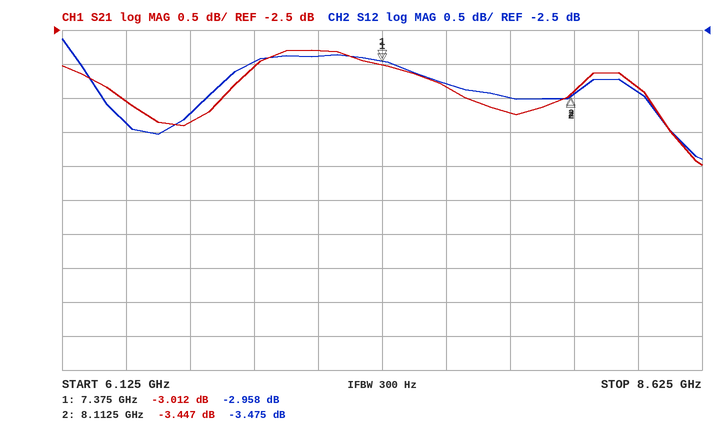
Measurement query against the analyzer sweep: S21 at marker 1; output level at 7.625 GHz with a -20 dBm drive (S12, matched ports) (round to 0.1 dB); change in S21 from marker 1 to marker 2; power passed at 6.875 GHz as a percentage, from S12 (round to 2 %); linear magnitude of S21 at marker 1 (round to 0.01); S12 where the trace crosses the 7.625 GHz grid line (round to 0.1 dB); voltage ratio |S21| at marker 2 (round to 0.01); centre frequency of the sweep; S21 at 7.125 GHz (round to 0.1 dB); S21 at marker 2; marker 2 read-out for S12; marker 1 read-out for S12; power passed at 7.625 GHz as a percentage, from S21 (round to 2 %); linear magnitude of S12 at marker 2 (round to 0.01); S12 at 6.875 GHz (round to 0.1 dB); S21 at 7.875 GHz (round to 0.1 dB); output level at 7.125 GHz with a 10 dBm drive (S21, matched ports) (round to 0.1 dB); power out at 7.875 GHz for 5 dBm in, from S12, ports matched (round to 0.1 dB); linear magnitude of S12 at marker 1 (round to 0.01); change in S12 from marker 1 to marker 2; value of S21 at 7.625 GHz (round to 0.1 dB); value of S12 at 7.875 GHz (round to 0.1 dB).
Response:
-3.012 dB
-23.3 dBm
-0.435 dB
50 %
0.71
-3.3 dB
0.67
7.375 GHz
-2.8 dB
-3.447 dB
-3.475 dB
-2.958 dB
46 %
0.67
-3.0 dB
-3.7 dB
7.2 dBm
1.5 dBm
0.71
-0.517 dB
-3.3 dB
-3.5 dB
